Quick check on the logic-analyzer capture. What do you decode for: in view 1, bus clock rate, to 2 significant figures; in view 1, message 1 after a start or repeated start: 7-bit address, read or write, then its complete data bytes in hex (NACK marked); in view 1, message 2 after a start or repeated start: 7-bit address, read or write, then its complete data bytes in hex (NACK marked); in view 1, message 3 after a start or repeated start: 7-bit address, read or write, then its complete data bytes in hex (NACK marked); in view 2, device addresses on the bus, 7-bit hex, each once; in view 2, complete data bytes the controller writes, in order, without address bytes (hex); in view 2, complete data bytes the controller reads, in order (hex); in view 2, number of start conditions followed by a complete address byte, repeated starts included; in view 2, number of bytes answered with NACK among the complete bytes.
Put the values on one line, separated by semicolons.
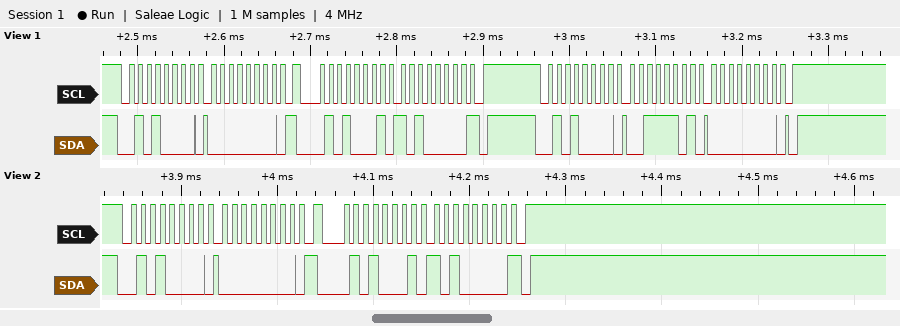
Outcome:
100 kHz; 0x28 write: 00; 0x28 read: A0 NACK; 0x28 write: 3D 00; 0x28; 00; A0; 2; 1
